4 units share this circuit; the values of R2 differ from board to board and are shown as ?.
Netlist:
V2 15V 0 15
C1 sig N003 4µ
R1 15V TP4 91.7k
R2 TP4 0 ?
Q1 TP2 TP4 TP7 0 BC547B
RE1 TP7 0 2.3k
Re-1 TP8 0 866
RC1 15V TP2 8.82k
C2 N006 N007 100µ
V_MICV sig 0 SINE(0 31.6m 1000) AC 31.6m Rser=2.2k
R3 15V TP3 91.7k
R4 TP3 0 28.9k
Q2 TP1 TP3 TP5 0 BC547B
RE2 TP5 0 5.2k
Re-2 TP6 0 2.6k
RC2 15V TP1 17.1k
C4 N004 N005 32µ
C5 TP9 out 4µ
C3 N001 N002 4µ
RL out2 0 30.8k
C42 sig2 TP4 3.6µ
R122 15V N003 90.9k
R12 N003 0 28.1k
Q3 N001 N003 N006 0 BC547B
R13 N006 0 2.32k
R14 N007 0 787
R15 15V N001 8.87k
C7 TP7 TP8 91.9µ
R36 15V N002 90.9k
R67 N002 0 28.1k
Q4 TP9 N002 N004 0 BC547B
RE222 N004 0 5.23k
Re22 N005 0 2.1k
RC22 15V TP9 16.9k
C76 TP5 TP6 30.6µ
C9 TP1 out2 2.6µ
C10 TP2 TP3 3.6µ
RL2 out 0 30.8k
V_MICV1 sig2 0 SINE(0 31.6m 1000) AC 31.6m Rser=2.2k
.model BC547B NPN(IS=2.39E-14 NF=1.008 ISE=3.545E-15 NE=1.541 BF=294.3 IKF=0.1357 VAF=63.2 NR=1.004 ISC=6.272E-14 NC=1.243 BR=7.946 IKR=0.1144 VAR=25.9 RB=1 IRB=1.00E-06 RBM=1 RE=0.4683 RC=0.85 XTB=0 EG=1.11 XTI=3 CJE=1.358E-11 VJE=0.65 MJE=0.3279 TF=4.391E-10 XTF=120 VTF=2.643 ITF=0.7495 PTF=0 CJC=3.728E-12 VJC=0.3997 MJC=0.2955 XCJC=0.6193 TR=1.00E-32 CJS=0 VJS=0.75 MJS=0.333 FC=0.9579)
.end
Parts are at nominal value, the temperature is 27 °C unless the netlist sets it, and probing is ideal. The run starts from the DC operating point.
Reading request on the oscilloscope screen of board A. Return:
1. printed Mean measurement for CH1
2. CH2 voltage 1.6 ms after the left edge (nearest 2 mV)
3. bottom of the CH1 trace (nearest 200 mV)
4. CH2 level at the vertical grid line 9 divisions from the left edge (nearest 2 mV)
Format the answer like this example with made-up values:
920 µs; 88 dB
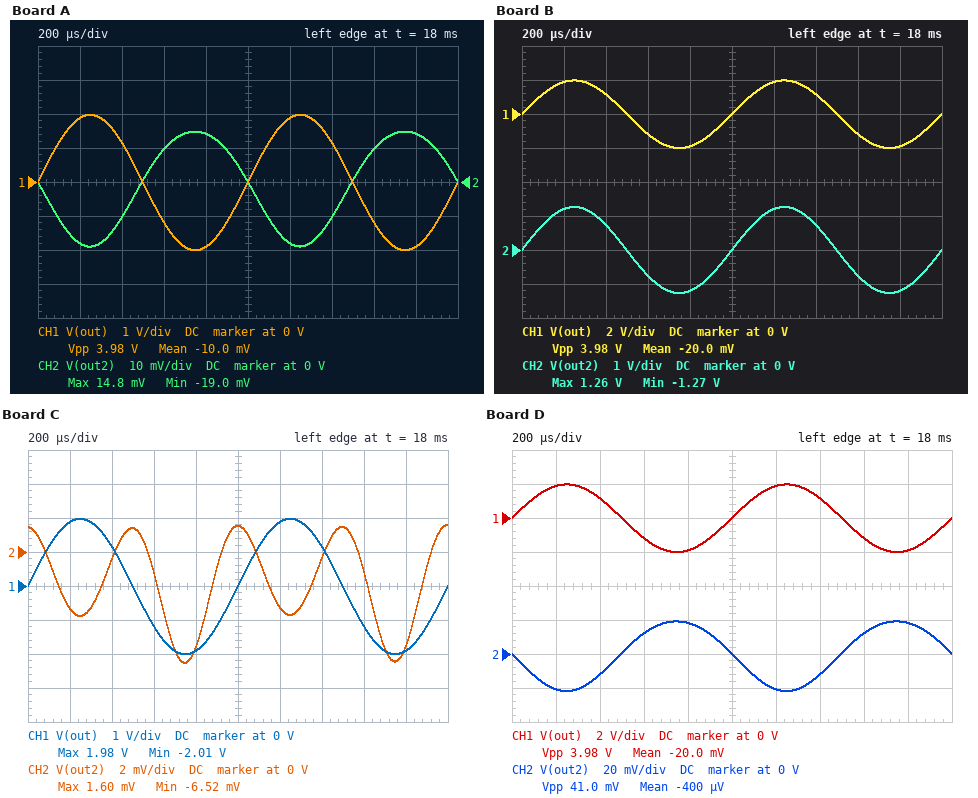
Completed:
-10.0 mV; 10 mV; -2.0 V; 14 mV
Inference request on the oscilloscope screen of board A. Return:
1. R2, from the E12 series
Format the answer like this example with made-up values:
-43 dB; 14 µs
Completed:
68 kΩ
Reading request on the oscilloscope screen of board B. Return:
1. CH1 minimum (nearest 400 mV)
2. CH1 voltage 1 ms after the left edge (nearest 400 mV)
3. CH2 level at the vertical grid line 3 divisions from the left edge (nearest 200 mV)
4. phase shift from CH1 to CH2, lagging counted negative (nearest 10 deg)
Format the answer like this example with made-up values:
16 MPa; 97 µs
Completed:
-2.0 V; 0 V; -800 mV; 0 deg
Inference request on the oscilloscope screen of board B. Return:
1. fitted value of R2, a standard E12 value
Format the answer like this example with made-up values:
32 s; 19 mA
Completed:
8.2 kΩ
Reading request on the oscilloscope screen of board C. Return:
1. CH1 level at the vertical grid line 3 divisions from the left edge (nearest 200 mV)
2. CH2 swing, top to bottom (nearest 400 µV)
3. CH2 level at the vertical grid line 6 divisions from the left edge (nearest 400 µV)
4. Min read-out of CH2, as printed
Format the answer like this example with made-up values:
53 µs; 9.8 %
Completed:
-1.2 V; 8.0 mV; -3.2 mV; -6.52 mV
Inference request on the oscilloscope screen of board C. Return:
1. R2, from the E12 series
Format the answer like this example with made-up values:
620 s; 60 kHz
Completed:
47 kΩ
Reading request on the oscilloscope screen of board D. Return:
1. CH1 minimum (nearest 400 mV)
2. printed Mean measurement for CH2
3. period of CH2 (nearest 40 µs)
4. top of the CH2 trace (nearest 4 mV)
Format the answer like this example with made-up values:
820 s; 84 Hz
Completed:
-2.0 V; -400 µV; 1.00 ms; 20 mV
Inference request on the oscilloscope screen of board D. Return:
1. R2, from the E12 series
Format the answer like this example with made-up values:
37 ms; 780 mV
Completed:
82 kΩ
